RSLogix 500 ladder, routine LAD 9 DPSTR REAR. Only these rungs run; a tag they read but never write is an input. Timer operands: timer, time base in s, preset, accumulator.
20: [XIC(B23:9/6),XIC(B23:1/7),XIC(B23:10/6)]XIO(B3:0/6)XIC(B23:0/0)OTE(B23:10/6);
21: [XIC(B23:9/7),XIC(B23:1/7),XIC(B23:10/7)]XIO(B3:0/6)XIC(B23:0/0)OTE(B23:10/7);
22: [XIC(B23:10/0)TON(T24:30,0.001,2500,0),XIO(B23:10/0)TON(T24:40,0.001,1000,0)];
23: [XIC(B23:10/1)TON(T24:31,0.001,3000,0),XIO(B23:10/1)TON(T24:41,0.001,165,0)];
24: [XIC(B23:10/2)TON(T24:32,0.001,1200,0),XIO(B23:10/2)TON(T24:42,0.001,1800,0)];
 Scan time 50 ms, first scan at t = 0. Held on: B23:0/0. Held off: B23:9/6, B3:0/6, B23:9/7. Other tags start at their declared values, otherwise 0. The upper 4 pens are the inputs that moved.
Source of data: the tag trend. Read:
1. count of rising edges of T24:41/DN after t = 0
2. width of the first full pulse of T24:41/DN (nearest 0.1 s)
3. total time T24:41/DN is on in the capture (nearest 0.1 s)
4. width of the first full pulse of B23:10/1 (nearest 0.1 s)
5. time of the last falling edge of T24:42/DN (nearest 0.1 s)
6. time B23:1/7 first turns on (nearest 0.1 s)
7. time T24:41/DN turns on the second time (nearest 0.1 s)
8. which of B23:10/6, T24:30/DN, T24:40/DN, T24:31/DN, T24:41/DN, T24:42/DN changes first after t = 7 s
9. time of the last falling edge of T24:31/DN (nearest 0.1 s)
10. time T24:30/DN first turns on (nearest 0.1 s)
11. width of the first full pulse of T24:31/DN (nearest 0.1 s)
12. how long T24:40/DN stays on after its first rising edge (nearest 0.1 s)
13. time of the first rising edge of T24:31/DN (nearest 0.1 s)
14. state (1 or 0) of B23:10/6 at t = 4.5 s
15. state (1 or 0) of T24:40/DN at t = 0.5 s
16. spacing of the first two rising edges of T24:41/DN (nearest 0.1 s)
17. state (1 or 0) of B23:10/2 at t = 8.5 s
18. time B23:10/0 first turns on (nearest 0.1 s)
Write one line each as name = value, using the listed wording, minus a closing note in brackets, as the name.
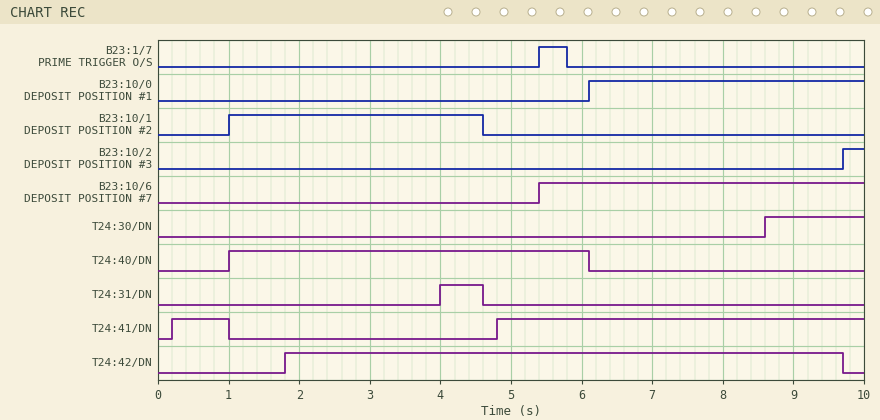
count of rising edges of T24:41/DN after t = 0 = 2
width of the first full pulse of T24:41/DN = 0.8 s
total time T24:41/DN is on in the capture = 6.0 s
width of the first full pulse of B23:10/1 = 3.6 s
time of the last falling edge of T24:42/DN = 9.7 s
time B23:1/7 first turns on = 5.4 s
time T24:41/DN turns on the second time = 4.8 s
which of B23:10/6, T24:30/DN, T24:40/DN, T24:31/DN, T24:41/DN, T24:42/DN changes first after t = 7 s = T24:30/DN
time of the last falling edge of T24:31/DN = 4.6 s
time T24:30/DN first turns on = 8.6 s
width of the first full pulse of T24:31/DN = 0.6 s
how long T24:40/DN stays on after its first rising edge = 5.1 s
time of the first rising edge of T24:31/DN = 4.0 s
state (1 or 0) of B23:10/6 at t = 4.5 s = 0
state (1 or 0) of T24:40/DN at t = 0.5 s = 0
spacing of the first two rising edges of T24:41/DN = 4.6 s
state (1 or 0) of B23:10/2 at t = 8.5 s = 0
time B23:10/0 first turns on = 6.1 s
